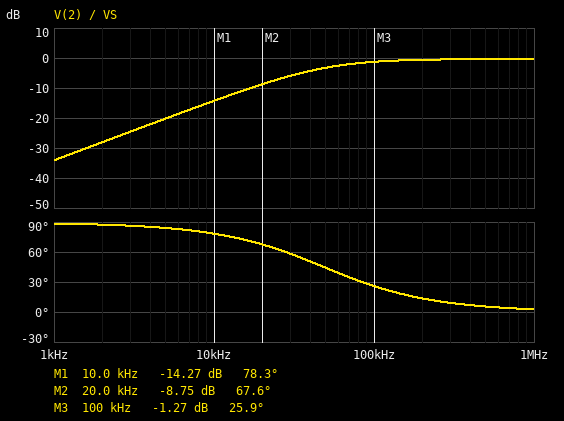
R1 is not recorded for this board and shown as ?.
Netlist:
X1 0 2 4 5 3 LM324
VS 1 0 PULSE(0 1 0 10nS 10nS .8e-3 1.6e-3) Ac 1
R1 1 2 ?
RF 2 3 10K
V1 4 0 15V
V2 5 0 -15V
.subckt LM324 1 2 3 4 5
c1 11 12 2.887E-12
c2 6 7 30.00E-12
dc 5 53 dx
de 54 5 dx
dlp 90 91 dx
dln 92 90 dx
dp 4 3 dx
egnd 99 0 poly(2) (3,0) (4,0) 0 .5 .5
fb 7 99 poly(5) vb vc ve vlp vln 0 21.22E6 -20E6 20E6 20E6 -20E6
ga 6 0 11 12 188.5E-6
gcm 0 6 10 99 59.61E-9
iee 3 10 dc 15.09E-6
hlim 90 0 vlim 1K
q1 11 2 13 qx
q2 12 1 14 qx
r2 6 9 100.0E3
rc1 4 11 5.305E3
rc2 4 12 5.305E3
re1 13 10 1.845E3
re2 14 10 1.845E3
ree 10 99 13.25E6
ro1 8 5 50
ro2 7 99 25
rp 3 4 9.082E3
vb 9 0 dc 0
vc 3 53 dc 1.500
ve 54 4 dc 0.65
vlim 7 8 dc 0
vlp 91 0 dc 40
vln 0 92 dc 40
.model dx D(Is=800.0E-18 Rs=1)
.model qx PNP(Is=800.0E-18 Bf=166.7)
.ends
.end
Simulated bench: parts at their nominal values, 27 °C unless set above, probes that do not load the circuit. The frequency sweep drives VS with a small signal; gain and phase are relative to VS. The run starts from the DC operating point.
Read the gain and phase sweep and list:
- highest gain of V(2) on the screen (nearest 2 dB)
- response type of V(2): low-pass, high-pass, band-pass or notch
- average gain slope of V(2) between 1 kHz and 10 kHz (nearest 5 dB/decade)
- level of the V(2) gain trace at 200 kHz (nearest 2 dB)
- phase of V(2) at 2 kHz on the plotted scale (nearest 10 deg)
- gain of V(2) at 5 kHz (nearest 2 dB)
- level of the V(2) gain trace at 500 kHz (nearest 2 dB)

0 dB
high-pass
20 dB/decade
0 dB
90 deg
-20 dB
0 dB
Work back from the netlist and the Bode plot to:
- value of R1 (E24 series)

510 Ω
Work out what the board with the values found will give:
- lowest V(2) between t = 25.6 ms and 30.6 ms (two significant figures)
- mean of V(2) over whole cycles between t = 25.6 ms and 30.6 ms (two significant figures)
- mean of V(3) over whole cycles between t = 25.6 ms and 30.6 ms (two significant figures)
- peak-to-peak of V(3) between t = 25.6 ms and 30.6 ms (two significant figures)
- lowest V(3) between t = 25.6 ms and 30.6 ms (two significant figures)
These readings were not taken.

-730 mV
110 mV
-7.5 V
15 V
-15 V
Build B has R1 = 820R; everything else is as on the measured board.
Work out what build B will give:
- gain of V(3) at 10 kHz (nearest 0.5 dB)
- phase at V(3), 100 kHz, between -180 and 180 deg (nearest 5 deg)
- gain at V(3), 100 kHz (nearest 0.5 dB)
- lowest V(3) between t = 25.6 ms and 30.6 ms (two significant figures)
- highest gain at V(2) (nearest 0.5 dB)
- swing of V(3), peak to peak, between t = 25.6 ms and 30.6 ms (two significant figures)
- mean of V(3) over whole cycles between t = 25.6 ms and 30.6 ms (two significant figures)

21.5 dB
125 deg
17.5 dB
-12 V
-0.5 dB
12 V
-6.1 V
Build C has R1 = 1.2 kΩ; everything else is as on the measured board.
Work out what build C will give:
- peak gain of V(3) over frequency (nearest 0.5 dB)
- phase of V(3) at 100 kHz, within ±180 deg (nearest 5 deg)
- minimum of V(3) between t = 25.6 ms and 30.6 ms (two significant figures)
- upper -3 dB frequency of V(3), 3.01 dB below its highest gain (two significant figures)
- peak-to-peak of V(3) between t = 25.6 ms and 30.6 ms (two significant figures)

18.5 dB
135 deg
-8.3 V
110 kHz
8.3 V
